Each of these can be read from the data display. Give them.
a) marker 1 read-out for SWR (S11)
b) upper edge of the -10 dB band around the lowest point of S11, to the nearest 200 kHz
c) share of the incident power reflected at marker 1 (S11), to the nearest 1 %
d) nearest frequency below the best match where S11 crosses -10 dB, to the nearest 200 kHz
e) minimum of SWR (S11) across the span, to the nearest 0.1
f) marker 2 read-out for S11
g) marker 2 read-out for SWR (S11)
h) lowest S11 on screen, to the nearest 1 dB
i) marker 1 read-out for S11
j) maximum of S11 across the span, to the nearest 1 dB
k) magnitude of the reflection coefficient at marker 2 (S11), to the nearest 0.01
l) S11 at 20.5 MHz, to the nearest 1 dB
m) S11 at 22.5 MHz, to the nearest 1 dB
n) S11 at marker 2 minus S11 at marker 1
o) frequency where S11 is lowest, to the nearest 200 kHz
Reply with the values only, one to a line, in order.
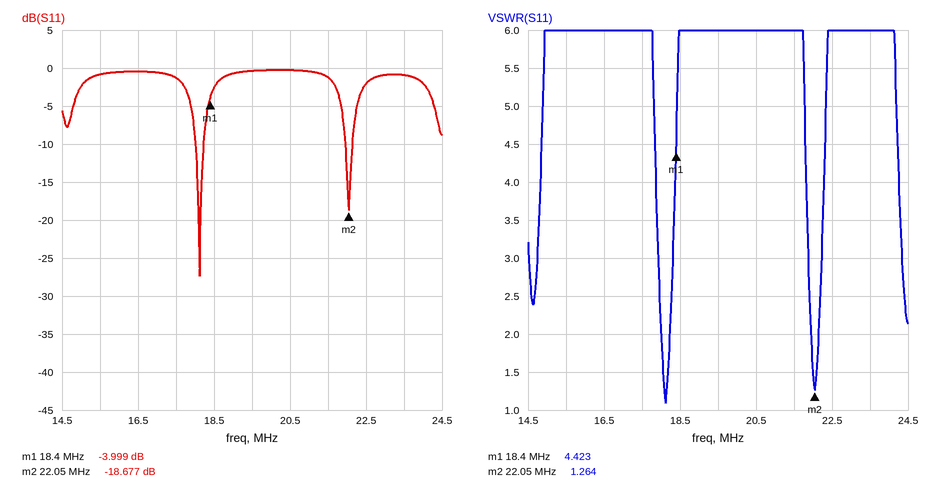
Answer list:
4.423
18.2 MHz
40 %
18.0 MHz
1.1
-18.677 dB
1.264
-27 dB
-3.999 dB
0 dB
0.12
0 dB
-2 dB
-14.678 dB
18.2 MHz
